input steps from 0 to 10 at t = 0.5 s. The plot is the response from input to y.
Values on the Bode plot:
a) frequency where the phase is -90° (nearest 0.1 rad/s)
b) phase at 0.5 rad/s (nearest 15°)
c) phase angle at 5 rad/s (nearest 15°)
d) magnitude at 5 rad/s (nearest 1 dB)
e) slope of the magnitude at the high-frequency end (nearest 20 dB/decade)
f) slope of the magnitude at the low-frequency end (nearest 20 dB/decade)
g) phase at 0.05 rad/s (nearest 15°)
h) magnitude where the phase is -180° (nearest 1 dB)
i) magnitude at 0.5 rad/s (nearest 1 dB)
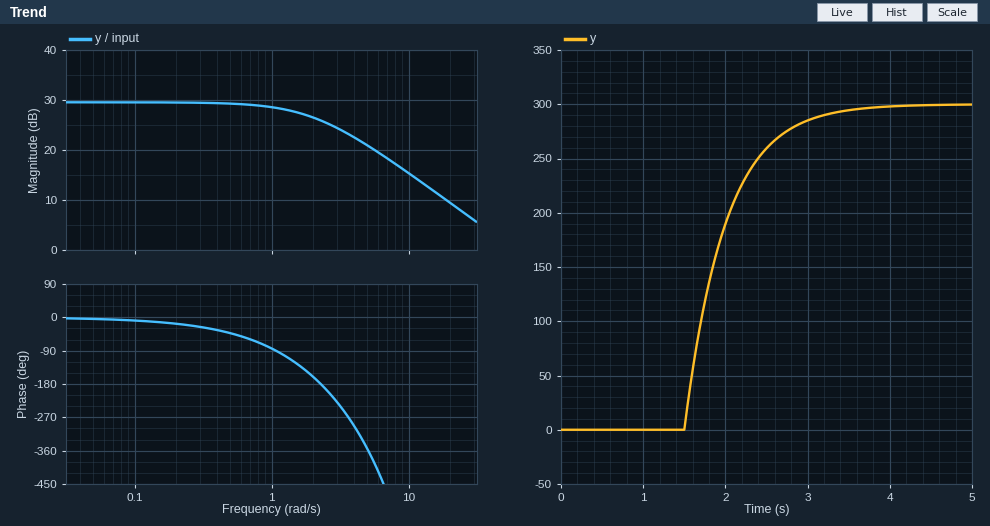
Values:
1.1 rad/s
-45°
-360°
21 dB
-20 dB/decade
0 dB/decade
0°
26 dB
29 dB
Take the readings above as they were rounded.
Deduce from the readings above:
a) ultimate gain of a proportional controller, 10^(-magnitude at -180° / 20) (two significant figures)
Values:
0.050
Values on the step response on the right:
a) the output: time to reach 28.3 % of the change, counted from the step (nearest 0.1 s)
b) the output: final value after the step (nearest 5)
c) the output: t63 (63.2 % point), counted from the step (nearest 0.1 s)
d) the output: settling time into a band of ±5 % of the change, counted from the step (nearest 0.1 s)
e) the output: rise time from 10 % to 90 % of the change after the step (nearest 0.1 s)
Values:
1.2 s
300
1.5 s
2.5 s
1.1 s
